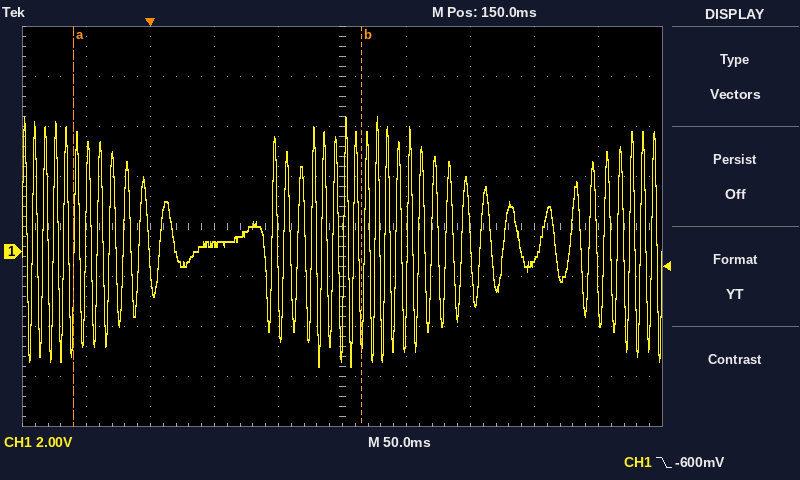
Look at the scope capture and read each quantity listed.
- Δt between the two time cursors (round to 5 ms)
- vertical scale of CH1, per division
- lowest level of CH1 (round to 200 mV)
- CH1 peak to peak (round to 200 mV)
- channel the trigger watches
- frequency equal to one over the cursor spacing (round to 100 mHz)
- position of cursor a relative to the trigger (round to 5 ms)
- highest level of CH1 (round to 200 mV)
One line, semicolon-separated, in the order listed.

225 ms; 2 V; -4.6 V; 10.0 V; CH1; 4.4 Hz; -60 ms; 5.4 V
